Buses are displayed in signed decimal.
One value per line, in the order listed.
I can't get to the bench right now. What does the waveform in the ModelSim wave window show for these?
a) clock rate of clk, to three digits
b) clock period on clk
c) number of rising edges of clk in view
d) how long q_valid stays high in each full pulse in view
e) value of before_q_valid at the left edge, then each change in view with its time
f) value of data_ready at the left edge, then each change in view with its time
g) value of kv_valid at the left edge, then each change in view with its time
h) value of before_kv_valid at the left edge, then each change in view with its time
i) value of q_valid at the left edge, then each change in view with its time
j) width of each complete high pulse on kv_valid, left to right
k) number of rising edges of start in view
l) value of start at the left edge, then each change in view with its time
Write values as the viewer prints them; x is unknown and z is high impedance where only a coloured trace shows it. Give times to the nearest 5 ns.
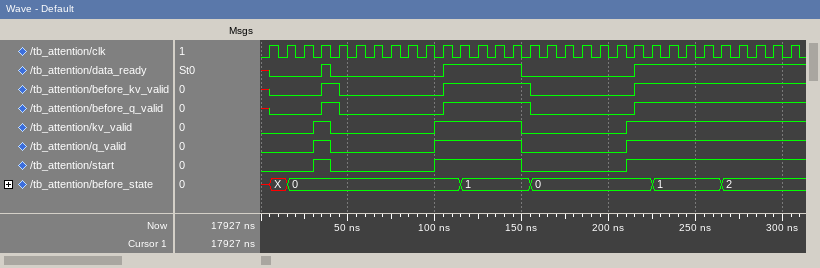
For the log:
100 MHz
10 ns
31
10 ns, 50 ns
x, 0 at 5 ns, 1 at 35 ns, 0 at 45 ns, 1 at 105 ns, 0 at 155 ns, 1 at 215 ns
x, 0 at 5 ns, 1 at 35 ns, 0 at 40 ns, 1 at 105 ns, 0 at 150 ns, 1 at 215 ns
0, 1 at 30 ns, 0 at 40 ns, 1 at 100 ns, 0 at 150 ns, 1 at 210 ns
x, 0 at 5 ns, 1 at 35 ns, 0 at 45 ns, 1 at 105 ns, 0 at 155 ns, 1 at 215 ns
0, 1 at 30 ns, 0 at 40 ns, 1 at 100 ns, 0 at 150 ns, 1 at 210 ns
10 ns, 50 ns
3
0, 1 at 30 ns, 0 at 40 ns, 1 at 100 ns, 0 at 150 ns, 1 at 210 ns
